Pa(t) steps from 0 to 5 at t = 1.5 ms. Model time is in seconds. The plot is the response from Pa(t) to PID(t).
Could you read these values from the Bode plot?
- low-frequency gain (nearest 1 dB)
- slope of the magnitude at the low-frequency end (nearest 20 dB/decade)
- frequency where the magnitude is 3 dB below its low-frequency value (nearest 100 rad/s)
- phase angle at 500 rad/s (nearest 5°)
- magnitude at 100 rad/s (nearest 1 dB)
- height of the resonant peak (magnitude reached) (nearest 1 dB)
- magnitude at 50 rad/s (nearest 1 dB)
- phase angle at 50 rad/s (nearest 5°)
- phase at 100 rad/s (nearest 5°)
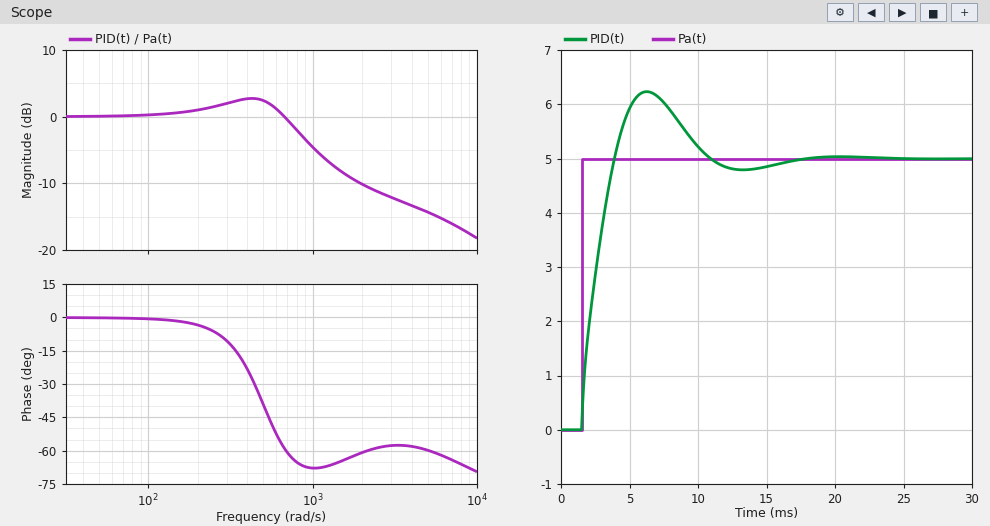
0 dB
0 dB/decade
900 rad/s
-40°
0 dB
3 dB
0 dB
0°
0°
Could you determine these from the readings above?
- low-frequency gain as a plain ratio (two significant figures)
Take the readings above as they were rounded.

1.0
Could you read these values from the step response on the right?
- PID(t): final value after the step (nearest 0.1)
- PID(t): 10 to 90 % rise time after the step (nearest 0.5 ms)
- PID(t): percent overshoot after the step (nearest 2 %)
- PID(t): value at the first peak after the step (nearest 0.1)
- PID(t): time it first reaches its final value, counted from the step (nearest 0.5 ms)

5.0
2.0 ms
24 %
6.2
2.5 ms
